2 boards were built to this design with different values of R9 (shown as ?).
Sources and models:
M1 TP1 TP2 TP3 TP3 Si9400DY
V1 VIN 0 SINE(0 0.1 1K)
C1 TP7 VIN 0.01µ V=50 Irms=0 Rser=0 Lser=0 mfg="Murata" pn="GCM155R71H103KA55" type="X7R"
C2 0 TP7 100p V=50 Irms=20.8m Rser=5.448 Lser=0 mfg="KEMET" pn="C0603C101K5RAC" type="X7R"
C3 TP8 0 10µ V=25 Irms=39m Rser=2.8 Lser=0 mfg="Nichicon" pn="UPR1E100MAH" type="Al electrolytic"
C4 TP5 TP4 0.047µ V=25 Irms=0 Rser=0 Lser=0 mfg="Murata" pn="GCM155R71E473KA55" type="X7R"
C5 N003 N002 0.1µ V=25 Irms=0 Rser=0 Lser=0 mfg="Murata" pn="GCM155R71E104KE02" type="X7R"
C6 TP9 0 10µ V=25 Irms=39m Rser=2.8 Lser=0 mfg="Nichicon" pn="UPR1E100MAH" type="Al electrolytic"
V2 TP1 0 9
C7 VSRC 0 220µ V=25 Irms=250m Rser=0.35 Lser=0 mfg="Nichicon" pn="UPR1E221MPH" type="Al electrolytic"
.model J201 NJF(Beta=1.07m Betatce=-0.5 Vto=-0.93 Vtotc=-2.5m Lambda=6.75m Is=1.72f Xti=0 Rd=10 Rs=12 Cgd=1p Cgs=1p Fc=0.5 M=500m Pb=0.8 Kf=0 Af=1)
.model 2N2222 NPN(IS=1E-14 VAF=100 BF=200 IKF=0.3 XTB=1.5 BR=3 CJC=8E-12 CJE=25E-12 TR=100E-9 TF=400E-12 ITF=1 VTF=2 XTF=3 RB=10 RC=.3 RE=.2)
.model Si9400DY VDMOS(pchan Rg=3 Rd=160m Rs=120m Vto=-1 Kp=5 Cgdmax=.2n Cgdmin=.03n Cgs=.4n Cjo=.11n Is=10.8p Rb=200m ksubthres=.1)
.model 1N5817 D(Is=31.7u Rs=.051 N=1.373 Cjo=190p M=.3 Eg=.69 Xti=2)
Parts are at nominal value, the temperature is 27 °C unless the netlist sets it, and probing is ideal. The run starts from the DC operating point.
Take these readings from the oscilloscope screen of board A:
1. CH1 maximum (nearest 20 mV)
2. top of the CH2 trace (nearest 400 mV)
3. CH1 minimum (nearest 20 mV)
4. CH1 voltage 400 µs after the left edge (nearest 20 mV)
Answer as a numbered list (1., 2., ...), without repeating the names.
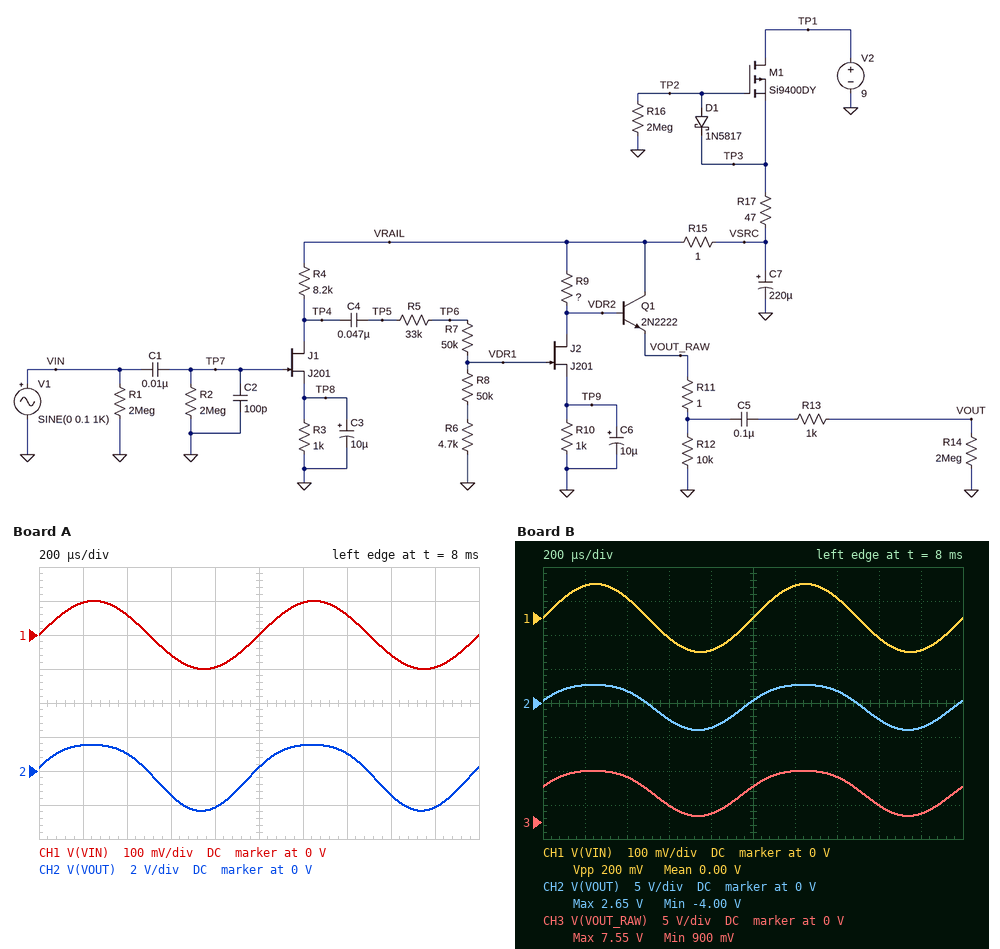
1. 100 mV
2. 1.6 V
3. -100 mV
4. 60 mV
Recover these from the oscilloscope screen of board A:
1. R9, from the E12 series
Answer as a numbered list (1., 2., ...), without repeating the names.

1. 4.7 kΩ
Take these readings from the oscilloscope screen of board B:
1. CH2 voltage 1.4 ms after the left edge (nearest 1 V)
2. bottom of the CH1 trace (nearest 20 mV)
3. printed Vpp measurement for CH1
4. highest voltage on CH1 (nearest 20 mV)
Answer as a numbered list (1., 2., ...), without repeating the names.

1. 2 V
2. -100 mV
3. 200 mV
4. 100 mV
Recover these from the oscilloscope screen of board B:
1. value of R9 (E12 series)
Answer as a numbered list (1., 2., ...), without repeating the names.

1. 8.2 kΩ
